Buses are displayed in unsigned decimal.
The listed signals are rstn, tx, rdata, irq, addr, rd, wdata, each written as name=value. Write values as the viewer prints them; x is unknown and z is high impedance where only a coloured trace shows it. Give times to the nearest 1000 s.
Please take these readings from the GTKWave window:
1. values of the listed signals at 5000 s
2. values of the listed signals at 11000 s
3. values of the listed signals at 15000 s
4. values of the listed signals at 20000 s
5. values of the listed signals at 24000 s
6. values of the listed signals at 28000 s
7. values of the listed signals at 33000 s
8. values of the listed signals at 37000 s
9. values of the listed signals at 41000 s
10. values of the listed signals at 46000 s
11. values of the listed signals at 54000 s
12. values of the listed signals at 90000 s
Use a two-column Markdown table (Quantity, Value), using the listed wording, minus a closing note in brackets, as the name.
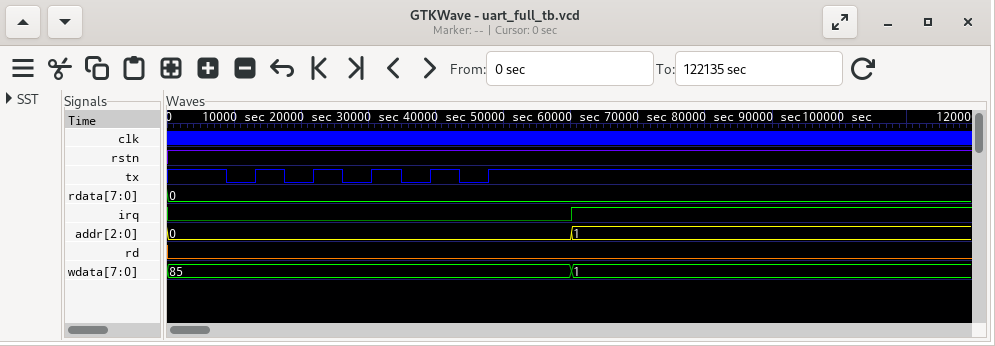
| Quantity | Value |
|---|---|
| values of the listed signals at 5000 s | rstn=1, tx=1, rdata=0, irq=0, addr=0, rd=0, wdata=85 |
| values of the listed signals at 11000 s | rstn=1, tx=0, rdata=0, irq=0, addr=0, rd=0, wdata=85 |
| values of the listed signals at 15000 s | rstn=1, tx=1, rdata=0, irq=0, addr=0, rd=0, wdata=85 |
| values of the listed signals at 20000 s | rstn=1, tx=0, rdata=0, irq=0, addr=0, rd=0, wdata=85 |
| values of the listed signals at 24000 s | rstn=1, tx=1, rdata=0, irq=0, addr=0, rd=0, wdata=85 |
| values of the listed signals at 28000 s | rstn=1, tx=0, rdata=0, irq=0, addr=0, rd=0, wdata=85 |
| values of the listed signals at 33000 s | rstn=1, tx=1, rdata=0, irq=0, addr=0, rd=0, wdata=85 |
| values of the listed signals at 37000 s | rstn=1, tx=0, rdata=0, irq=0, addr=0, rd=0, wdata=85 |
| values of the listed signals at 41000 s | rstn=1, tx=1, rdata=0, irq=0, addr=0, rd=0, wdata=85 |
| values of the listed signals at 46000 s | rstn=1, tx=0, rdata=0, irq=0, addr=0, rd=0, wdata=85 |
| values of the listed signals at 54000 s | rstn=1, tx=1, rdata=0, irq=0, addr=0, rd=0, wdata=85 |
| values of the listed signals at 90000 s | rstn=1, tx=1, rdata=0, irq=1, addr=1, rd=0, wdata=1 |
